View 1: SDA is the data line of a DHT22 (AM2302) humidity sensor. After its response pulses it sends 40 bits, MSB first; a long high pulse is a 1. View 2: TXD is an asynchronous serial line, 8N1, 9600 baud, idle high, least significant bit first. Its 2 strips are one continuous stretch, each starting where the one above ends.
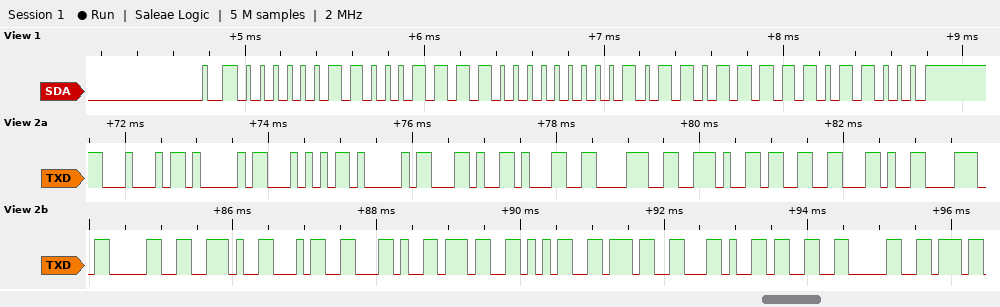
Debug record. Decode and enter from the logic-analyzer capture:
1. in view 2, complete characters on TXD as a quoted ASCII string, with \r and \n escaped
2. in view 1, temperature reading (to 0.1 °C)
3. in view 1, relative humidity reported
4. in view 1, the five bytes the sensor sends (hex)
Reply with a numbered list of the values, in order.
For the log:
1. "DATA,18.3,80.4,757,30"
2. 18.3 °C
3. 79.8 %
4. 03 1E 00 B7 D8
